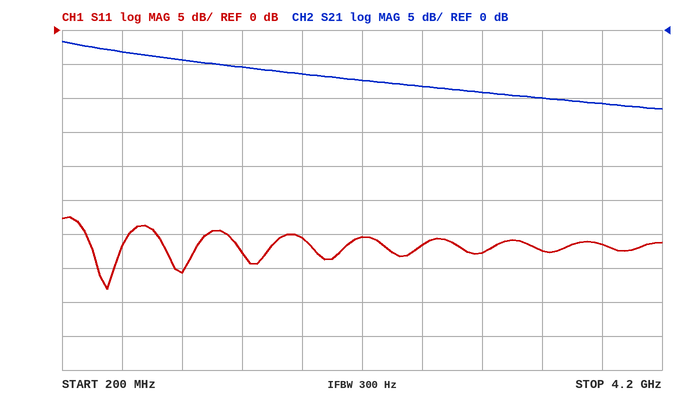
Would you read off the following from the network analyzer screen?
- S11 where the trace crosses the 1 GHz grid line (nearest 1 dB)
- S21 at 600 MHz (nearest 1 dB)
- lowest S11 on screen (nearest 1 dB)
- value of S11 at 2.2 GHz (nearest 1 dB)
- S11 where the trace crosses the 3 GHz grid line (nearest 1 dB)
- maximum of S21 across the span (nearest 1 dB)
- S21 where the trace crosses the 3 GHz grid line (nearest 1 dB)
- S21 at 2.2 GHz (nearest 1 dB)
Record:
-36 dB
-3 dB
-38 dB
-30 dB
-33 dB
-2 dB
-9 dB
-7 dB
